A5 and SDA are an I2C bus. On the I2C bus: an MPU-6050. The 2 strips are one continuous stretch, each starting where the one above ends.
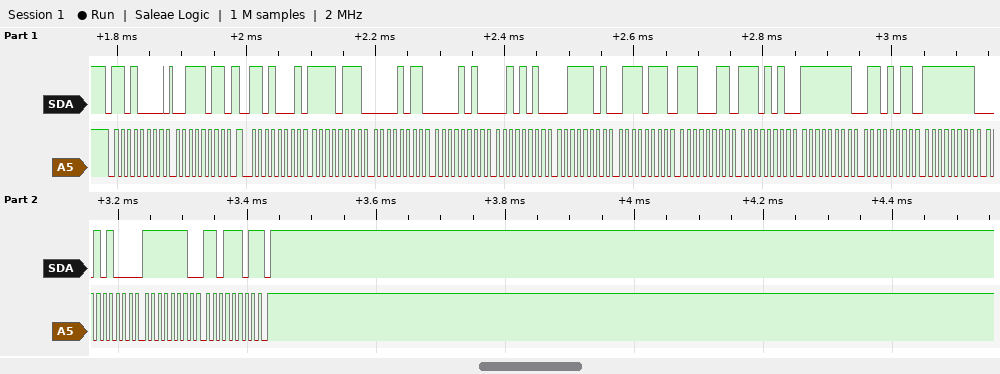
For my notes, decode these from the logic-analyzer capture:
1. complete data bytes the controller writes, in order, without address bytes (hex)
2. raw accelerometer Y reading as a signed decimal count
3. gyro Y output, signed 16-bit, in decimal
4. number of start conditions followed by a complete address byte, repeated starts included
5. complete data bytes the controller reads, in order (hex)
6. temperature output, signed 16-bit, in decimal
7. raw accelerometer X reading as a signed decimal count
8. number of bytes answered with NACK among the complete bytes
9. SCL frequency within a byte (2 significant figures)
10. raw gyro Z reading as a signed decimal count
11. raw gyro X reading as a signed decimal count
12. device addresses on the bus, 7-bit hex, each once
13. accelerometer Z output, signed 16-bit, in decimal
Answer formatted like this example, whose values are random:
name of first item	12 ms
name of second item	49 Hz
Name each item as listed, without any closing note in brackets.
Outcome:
complete data bytes the controller writes, in order, without address bytes	3B
raw accelerometer Y reading as a signed decimal count	2602
gyro Y output, signed 16-bit, in decimal	-216
number of start conditions followed by a complete address byte, repeated starts included	2
complete data bytes the controller reads, in order	F7 0B 0A 2A 3D 77 E3 EA FF 6B FF 28 FE DD
temperature output, signed 16-bit, in decimal	-7190
raw accelerometer X reading as a signed decimal count	-2293
number of bytes answered with NACK among the complete bytes	1
SCL frequency within a byte	100 kHz
raw gyro Z reading as a signed decimal count	-291
raw gyro X reading as a signed decimal count	-149
device addresses on the bus, 7-bit hex, each once	0x68
accelerometer Z output, signed 16-bit, in decimal	15735
